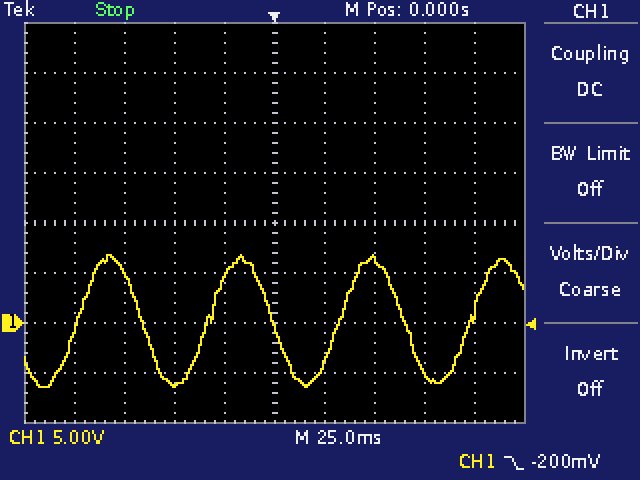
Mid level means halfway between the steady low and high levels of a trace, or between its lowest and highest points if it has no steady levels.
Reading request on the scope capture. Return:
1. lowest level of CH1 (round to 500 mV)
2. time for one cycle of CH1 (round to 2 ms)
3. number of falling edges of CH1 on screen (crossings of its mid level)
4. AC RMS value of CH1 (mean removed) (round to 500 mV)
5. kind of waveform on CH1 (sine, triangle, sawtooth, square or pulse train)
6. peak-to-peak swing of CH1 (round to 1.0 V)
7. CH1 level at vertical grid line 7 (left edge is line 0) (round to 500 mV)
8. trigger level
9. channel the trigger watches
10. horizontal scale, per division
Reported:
-6.5 V
66 ms
3
4.5 V
sine
13.0 V
6.5 V
-200 mV
CH1
25 ms
